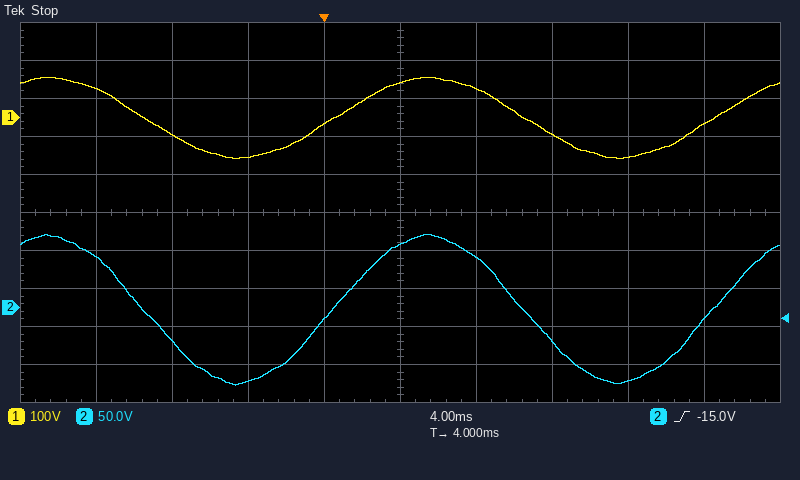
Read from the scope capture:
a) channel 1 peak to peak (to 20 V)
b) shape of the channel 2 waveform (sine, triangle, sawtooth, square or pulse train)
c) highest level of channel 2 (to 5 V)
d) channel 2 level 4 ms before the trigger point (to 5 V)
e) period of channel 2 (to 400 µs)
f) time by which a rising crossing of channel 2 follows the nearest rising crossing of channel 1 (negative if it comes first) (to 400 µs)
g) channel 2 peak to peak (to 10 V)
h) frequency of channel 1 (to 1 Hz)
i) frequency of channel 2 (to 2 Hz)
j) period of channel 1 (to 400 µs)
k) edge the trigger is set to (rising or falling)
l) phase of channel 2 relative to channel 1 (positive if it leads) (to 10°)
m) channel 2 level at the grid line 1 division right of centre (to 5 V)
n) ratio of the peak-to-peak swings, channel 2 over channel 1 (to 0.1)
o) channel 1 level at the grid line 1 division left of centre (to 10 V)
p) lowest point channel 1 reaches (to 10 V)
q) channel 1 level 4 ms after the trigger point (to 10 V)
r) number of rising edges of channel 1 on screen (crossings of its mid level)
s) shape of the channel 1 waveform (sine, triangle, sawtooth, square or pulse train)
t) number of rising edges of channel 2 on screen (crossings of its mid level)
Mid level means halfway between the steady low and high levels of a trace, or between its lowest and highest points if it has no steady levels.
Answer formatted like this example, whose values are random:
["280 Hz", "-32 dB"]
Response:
["220 V", "sine", "95 V", "-95 V", "20.0 ms", "0.0 ms", "200 V", "50 Hz", "50 Hz", "20.0 ms", "rising", "0°", "65 V", "0.9", "-20 V", "-110 V", "90 V", "2", "sine", "2"]
